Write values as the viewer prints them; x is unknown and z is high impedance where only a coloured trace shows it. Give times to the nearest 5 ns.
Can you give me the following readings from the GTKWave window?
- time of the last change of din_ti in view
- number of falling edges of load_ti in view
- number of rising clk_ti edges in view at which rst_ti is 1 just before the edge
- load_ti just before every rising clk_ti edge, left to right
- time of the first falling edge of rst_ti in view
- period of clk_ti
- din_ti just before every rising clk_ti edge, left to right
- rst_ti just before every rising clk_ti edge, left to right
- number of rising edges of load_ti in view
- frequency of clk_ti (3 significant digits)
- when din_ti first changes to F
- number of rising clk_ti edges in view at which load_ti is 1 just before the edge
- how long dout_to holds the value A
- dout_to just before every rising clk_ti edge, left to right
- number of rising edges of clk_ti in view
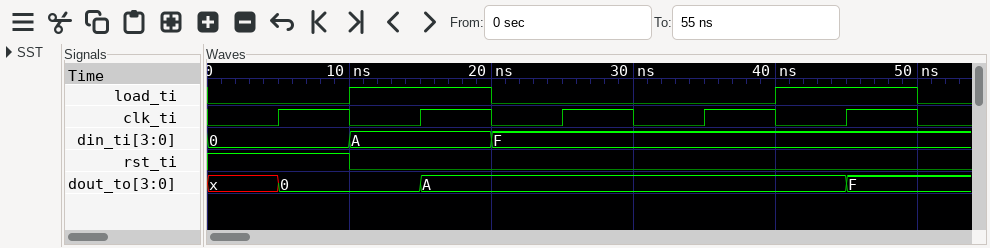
20 ns
2
1
0 1 0 0 1
10 ns
10 ns
0, A, F, F, F
1 0 0 0 0
2
100 MHz
20 ns
2
30 ns
x, 0, A, A, A
5
